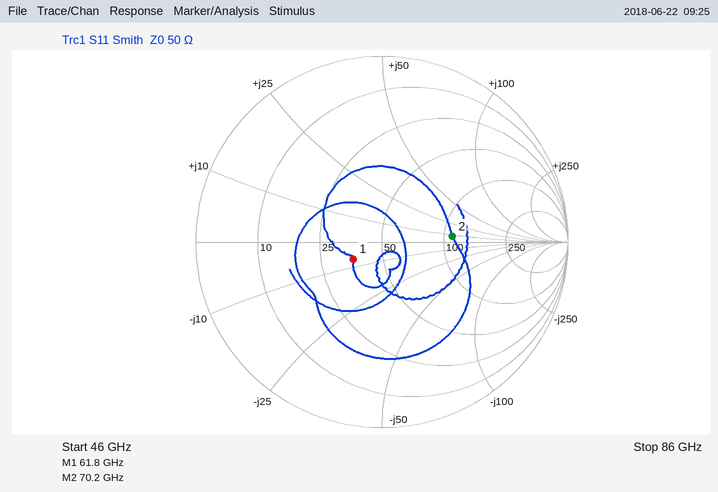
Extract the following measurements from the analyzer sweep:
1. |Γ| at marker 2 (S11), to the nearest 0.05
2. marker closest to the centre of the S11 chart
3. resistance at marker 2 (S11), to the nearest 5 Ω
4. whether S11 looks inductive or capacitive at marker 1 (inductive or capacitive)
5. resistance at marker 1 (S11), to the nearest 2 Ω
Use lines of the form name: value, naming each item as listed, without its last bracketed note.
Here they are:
|Γ| at marker 2 (S11), to the nearest 0.05: 0.40
marker closest to the centre of the S11 chart: marker 1
resistance at marker 2 (S11), to the nearest 5 Ω: 110 Ω
whether S11 looks inductive or capacitive at marker 1: capacitive
resistance at marker 1 (S11), to the nearest 2 Ω: 36 Ω
